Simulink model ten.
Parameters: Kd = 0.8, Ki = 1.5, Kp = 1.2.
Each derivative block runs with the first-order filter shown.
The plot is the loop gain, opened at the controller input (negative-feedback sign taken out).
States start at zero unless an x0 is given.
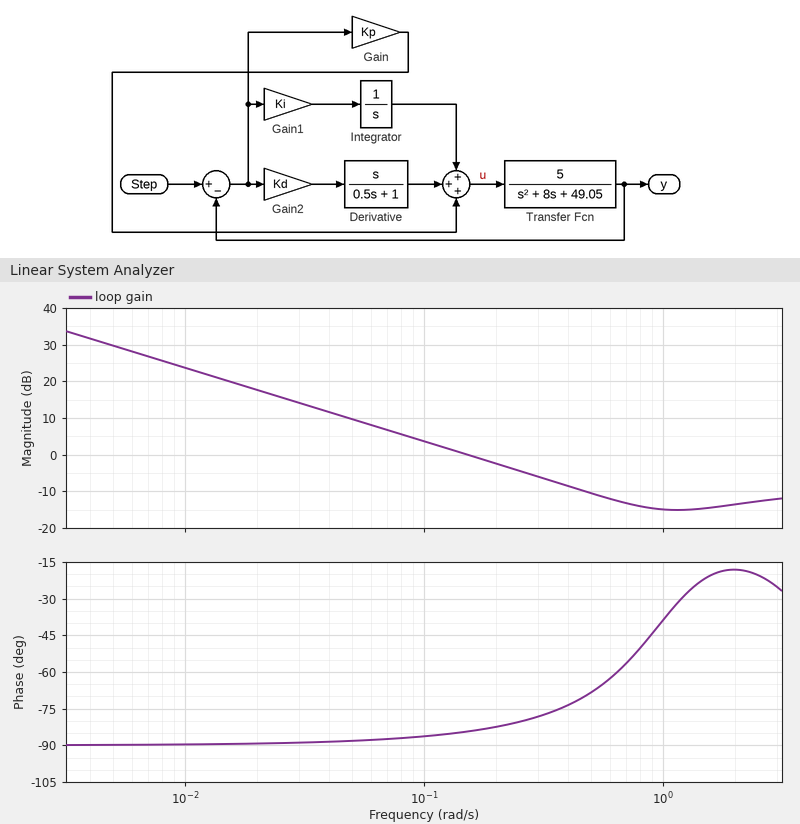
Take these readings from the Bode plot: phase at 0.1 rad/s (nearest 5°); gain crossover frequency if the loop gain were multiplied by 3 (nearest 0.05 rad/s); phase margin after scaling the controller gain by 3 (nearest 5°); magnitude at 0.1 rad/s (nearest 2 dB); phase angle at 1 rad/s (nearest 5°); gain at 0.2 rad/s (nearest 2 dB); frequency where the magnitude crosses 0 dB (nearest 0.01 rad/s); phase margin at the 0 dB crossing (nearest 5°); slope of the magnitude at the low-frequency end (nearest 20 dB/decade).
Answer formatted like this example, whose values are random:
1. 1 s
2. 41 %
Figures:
1. -85°
2. 0.45 rad/s
3. 110°
4. 4 dB
5. -40°
6. -2 dB
7. 0.15 rad/s
8. 95°
9. -20 dB/decade
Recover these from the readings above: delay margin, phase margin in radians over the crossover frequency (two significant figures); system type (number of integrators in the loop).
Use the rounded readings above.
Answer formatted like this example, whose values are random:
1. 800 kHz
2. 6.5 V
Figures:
1. 11 s
2. 1
